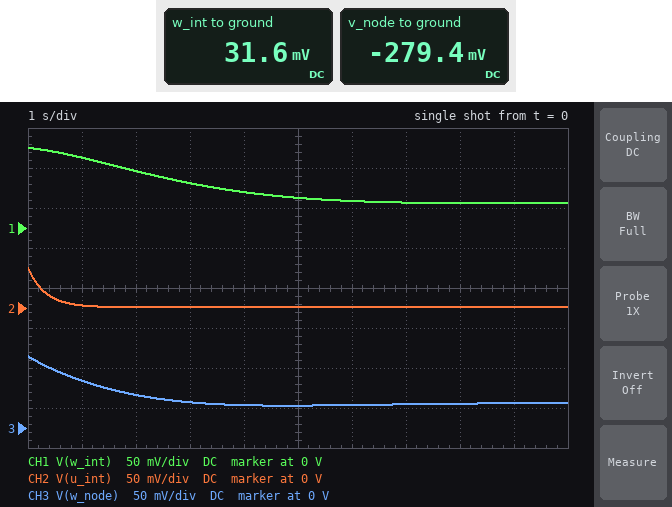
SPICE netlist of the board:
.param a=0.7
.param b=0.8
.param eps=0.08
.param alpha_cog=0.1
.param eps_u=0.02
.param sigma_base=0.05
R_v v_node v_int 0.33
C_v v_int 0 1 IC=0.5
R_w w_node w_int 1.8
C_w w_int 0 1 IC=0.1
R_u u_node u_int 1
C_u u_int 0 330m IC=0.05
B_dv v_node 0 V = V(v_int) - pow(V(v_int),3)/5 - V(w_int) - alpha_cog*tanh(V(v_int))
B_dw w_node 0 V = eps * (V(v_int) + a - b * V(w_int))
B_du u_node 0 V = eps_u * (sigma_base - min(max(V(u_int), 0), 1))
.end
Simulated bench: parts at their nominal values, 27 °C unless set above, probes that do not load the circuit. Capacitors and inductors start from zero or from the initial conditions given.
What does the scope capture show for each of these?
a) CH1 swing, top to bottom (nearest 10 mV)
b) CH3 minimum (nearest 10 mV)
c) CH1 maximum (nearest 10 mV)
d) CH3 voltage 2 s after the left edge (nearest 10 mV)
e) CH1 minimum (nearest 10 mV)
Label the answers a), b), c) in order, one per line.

a) 70 mV
b) 30 mV
c) 100 mV
d) 40 mV
e) 30 mV
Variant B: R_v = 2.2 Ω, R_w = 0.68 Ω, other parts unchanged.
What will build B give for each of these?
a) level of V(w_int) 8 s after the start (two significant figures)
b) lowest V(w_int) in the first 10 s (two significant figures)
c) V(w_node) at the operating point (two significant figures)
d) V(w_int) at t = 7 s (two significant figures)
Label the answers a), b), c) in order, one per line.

a) 62 mV
b) 57 mV
c) 32 mV
d) 65 mV
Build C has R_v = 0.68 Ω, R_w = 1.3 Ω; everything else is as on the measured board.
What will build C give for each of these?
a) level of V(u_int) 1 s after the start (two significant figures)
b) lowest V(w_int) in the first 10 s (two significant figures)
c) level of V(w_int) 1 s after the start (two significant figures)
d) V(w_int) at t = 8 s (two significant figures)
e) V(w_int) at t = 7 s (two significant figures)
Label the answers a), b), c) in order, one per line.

a) 3.2 mV
b) 35 mV
c) 89 mV
d) 38 mV
e) 41 mV
